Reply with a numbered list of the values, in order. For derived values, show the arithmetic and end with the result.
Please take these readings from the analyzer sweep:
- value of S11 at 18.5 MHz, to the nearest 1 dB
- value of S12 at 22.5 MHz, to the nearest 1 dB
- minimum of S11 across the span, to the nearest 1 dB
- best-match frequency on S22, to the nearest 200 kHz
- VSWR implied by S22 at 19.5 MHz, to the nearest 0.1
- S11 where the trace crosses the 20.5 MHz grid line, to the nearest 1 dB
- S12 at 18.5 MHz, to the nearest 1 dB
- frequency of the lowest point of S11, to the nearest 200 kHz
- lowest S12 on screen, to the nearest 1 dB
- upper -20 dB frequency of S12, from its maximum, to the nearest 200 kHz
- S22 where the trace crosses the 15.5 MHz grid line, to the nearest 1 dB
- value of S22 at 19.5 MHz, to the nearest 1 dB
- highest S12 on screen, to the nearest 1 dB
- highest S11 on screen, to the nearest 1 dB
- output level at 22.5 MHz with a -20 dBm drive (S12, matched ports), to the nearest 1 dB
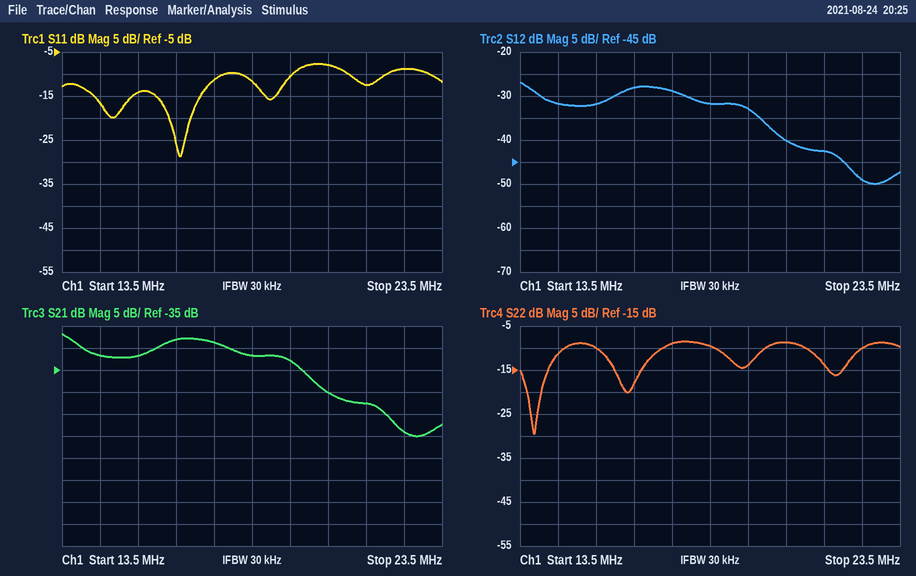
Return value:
1. -12 dB
2. -49 dB
3. -29 dB
4. 13.8 MHz
5. |Γ| = 10^(-14/20) = 0.1995; VSWR = (1 + 0.1995)/(1 − 0.1995) ≈ 1.5
6. -8 dB
7. -32 dB
8. 16.6 MHz
9. -50 dB
10. 22.2 MHz
11. -10 dB
12. -14 dB
13. -27 dB
14. -8 dB
15. -20 dBm + (-49 dB) = -69 dBm
